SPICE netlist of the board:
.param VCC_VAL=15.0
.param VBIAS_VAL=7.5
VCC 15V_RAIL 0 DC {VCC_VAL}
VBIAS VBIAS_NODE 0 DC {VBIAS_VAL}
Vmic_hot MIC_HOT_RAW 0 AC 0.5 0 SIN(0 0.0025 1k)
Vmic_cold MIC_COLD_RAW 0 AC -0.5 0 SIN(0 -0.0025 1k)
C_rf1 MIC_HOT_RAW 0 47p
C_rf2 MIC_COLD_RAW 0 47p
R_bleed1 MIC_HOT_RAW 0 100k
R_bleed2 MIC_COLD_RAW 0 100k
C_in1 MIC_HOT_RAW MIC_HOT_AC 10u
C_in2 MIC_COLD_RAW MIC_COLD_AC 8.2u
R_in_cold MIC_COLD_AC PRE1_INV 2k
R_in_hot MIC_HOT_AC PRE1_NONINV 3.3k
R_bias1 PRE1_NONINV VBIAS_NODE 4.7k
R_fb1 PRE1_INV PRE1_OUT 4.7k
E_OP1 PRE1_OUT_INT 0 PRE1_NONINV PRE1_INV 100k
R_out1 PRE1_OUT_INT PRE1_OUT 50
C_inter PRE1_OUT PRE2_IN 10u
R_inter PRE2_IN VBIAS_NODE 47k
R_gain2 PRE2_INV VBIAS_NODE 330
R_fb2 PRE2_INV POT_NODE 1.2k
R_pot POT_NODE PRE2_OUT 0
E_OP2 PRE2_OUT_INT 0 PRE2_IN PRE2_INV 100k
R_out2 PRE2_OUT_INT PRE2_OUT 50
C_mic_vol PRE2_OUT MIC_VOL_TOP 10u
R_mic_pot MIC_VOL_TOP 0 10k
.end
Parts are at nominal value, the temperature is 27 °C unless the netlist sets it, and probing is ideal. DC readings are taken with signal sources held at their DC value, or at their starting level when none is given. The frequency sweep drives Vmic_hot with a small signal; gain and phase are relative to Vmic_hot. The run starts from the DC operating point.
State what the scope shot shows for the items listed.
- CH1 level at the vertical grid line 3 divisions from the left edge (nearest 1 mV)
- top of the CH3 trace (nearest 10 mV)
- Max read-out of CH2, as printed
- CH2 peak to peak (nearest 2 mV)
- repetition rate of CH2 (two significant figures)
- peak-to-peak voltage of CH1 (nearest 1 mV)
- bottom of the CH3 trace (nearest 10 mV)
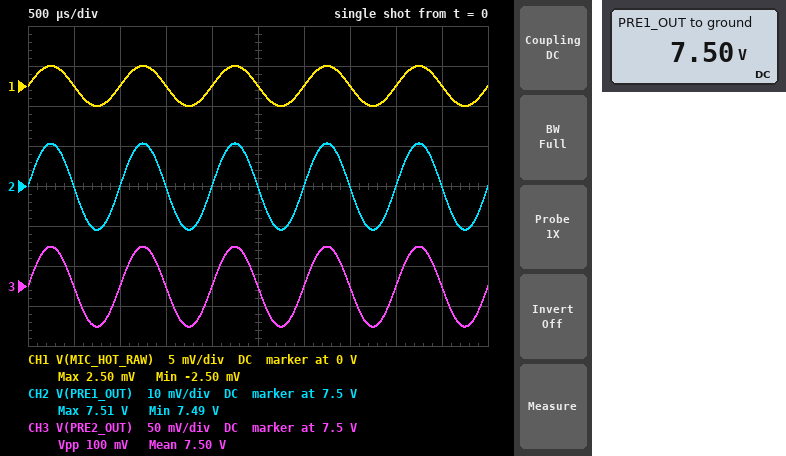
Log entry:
0 V
7.55 V
7.51 V
22 mV
1.0 kHz
5 mV
7.45 V
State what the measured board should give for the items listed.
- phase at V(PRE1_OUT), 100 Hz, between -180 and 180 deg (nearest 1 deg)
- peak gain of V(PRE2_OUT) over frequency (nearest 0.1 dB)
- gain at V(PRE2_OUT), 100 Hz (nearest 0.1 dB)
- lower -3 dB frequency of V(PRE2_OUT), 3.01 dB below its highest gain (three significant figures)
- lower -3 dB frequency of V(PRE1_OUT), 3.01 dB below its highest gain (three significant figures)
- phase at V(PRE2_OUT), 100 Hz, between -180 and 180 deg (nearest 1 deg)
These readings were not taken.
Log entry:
5 deg
23.3 dB
23.2 dB
9.46 Hz
9.45 Hz
5 deg
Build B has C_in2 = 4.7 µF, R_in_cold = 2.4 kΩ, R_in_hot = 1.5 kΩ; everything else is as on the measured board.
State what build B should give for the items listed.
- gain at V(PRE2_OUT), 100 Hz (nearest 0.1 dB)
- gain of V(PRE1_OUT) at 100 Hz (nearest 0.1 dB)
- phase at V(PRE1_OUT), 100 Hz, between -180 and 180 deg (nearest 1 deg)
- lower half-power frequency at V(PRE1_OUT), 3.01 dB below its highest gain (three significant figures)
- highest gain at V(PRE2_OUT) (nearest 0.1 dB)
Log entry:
23.4 dB
10.1 dB
7 deg
13.4 Hz
23.5 dB
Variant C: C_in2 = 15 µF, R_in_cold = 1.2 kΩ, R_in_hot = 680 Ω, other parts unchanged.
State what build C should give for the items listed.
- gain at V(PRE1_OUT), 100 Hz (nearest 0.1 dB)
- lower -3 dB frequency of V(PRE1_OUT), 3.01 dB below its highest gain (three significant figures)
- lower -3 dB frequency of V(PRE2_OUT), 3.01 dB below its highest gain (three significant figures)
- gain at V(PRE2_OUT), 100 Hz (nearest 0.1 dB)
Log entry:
15.9 dB
9.25 Hz
9.26 Hz
29.2 dB
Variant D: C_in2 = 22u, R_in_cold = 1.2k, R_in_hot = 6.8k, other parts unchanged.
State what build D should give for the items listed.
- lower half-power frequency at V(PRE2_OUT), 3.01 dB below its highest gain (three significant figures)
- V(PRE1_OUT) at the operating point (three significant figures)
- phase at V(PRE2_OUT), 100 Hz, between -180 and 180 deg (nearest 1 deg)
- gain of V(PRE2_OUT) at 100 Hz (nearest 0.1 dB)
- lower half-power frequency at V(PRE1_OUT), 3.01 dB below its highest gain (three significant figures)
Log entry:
6.08 Hz
7.50 V
4 deg
25.3 dB
6.06 Hz
